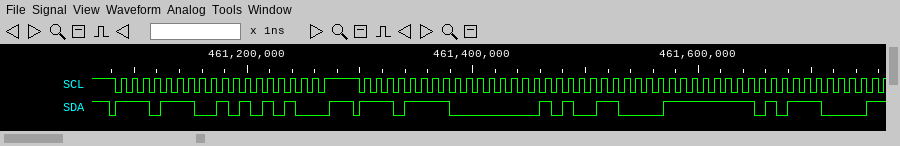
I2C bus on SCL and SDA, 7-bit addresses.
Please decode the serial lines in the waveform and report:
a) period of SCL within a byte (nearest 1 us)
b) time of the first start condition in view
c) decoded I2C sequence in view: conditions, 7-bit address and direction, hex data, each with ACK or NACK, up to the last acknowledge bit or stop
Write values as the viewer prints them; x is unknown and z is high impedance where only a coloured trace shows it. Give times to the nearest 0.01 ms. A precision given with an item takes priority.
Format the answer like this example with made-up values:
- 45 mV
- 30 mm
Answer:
- 10 us
- 461.08 ms
- start, address 77 write ACK, AA ACK, stop, start, address 77 read ACK, 01 ACK, 98 ACK, FF ACK, B8 ACK
